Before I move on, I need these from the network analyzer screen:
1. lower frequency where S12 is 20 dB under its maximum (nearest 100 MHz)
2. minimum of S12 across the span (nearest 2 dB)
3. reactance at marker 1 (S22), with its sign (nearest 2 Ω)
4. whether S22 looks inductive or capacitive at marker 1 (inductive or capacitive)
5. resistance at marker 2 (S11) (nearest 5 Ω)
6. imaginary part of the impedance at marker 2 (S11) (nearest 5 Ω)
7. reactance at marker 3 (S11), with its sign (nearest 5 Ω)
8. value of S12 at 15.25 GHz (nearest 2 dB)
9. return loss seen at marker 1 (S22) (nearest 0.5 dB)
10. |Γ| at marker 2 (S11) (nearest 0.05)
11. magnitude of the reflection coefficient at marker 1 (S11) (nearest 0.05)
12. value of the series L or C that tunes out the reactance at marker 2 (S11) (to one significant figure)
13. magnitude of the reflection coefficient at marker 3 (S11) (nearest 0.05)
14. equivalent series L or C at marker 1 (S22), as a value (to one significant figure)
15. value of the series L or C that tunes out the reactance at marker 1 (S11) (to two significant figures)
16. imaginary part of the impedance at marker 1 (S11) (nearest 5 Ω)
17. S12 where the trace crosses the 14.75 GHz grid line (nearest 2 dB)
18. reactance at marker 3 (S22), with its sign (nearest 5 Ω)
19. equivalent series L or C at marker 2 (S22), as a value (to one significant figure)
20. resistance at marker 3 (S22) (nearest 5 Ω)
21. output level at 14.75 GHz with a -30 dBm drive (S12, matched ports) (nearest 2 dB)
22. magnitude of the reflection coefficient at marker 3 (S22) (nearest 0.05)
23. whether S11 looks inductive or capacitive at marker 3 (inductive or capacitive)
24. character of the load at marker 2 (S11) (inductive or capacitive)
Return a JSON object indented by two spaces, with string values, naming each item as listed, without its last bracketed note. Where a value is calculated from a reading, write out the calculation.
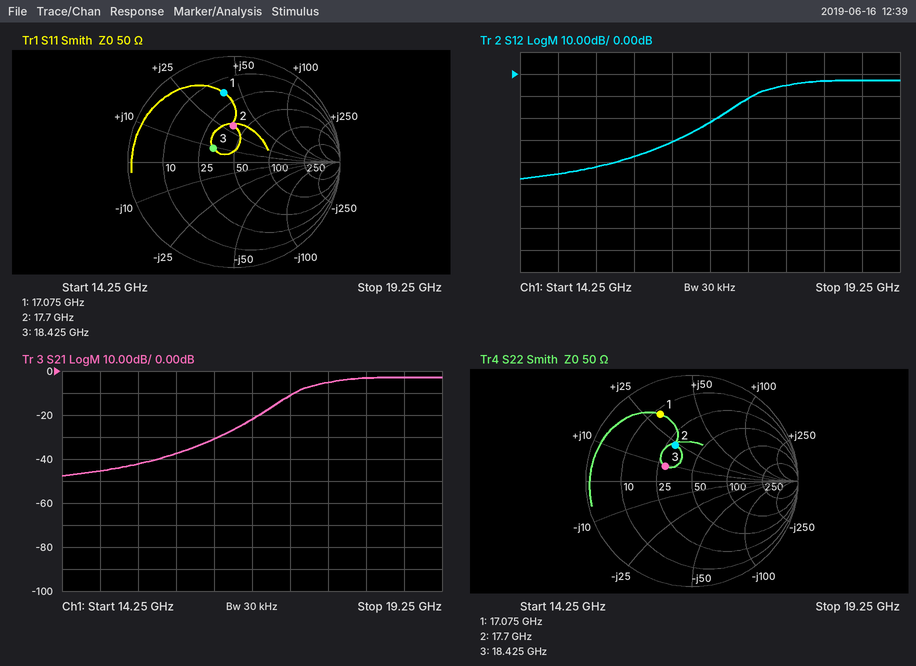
{
  "lower frequency where S12 is 20 dB under its maximum": "16.7 GHz",
  "minimum of S12 across the span": "-48 dB",
  "reactance at marker 1 (S22), with its sign": "+30 Ω",
  "whether S22 looks inductive or capacitive at marker 1": "inductive",
  "resistance at marker 2 (S11)": "40 Ω",
  "imaginary part of the impedance at marker 2 (S11)": "+30 Ω",
  "reactance at marker 3 (S11), with its sign": "+10 Ω",
  "value of S12 at 15.25 GHz": "-42 dB",
  "return loss seen at marker 1 (S22)": "3.0 dB",
  "|Γ| at marker 2 (S11)": "0.35",
  "magnitude of the reflection coefficient at marker 1 (S11)": "0.65",
  "value of the series L or C that tunes out the reactance at marker 2 (S11)": "C = 1/(2π × 17.7 GHz × 30 Ω) ≈ 300 fF",
  "magnitude of the reflection coefficient at marker 3 (S11)": "0.25",
  "equivalent series L or C at marker 1 (S22), as a value": "L = 30 Ω/(2π × 17.075 GHz) ≈ 280 pH, so 300 pH to one significant figure",
  "value of the series L or C that tunes out the reactance at marker 1 (S11)": "C = 1/(2π × 17.075 GHz × 40 Ω) ≈ 233 fF, so 230 fF to two significant figures",
  "imaginary part of the impedance at marker 1 (S11)": "+40 Ω",
  "S12 where the trace crosses the 14.75 GHz grid line": "-46 dB",
  "reactance at marker 3 (S22), with its sign": "+10 Ω",
  "equivalent series L or C at marker 2 (S22), as a value": "L = 25 Ω/(2π × 17.7 GHz) ≈ 225 pH, so 200 pH to one significant figure",
  "resistance at marker 3 (S22)": "30 Ω",
  "output level at 14.75 GHz with a -30 dBm drive (S12, matched ports)": "-30 dBm + (-46 dB) = -76 dBm",
  "magnitude of the reflection coefficient at marker 3 (S22)": "0.30",
  "whether S11 looks inductive or capacitive at marker 3": "inductive",
  "character of the load at marker 2 (S11)": "inductive"
}
